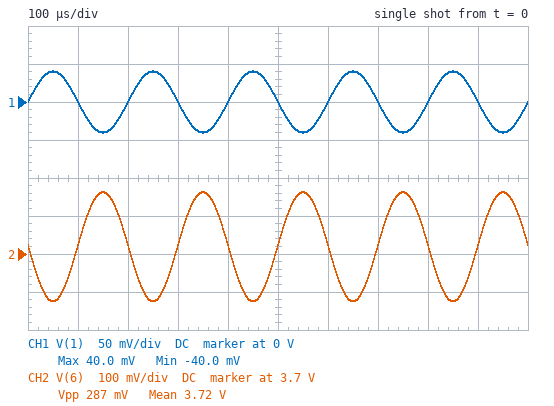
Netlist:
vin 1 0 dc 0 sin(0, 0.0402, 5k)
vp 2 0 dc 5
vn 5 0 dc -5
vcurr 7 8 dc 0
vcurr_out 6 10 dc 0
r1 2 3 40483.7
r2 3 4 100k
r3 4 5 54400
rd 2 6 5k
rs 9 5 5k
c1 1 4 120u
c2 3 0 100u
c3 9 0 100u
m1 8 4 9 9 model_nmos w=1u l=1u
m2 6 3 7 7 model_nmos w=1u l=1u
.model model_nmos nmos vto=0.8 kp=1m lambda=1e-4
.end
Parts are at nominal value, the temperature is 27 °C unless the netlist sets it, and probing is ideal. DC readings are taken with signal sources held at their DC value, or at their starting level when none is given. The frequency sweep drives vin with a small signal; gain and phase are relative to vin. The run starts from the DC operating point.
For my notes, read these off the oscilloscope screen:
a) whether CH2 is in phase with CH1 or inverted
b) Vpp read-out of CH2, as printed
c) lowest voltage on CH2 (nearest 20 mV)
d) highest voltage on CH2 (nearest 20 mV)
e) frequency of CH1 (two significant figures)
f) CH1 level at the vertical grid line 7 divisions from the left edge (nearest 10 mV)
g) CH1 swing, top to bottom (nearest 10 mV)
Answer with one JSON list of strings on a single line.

["inverted", "287 mV", "3.58 V", "3.86 V", "5.0 kHz", "0 V", "80 mV"]
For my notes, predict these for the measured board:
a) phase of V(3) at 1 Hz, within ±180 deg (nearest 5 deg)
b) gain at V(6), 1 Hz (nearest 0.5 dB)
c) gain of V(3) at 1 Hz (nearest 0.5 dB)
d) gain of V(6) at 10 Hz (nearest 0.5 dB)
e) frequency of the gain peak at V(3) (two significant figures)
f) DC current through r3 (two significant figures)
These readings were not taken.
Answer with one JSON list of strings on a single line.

["-85 deg", "6.5 dB", "-36.0 dB", "11.0 dB", "43 mHz", "51 µA"]
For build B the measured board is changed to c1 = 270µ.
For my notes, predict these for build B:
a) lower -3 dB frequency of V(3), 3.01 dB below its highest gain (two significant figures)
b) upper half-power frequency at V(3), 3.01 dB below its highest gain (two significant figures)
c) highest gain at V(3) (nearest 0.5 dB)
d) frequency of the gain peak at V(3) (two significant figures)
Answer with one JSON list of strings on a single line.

["10 mHz", "82 mHz", "-13.0 dB", "29 mHz"]
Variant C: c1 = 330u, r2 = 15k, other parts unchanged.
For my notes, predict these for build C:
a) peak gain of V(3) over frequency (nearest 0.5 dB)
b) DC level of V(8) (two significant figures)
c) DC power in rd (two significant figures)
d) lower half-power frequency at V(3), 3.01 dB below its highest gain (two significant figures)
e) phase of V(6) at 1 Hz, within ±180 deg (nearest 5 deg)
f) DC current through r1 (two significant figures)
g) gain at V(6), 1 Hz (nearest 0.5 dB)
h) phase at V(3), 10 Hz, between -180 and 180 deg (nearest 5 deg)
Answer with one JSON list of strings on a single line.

["-5.0 dB", "-590 mV", "1.9 mW", "13 mHz", "-130 deg", "91 µA", "8.0 dB", "-90 deg"]
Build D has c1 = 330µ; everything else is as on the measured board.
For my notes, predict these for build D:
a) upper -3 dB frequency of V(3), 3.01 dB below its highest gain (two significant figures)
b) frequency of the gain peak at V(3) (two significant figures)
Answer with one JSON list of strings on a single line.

["78 mHz", "26 mHz"]
